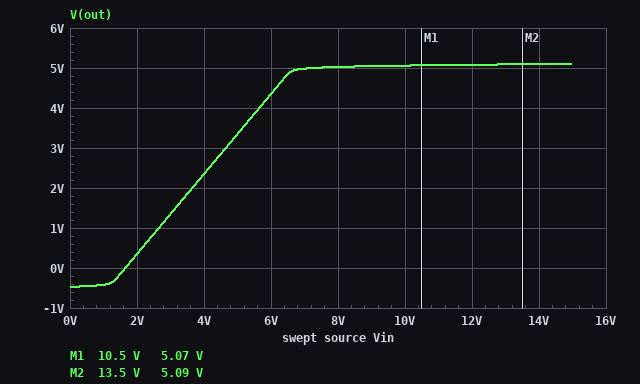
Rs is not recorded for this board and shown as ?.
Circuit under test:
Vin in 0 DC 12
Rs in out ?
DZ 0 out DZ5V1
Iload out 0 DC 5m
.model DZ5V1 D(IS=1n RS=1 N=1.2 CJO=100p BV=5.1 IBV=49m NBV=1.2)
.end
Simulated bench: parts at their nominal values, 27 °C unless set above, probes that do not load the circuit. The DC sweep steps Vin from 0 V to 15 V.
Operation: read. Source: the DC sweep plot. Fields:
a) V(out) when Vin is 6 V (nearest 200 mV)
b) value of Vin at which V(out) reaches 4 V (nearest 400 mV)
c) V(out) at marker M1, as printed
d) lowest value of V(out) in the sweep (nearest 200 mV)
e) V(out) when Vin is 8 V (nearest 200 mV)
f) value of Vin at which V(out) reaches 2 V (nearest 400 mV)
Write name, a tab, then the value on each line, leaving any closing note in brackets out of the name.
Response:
V(out) when Vin is 6 V	4.4 V
value of Vin at which V(out) reaches 4 V	5.6 V
V(out) at marker M1, as printed	5.07 V
lowest value of V(out) in the sweep	-400 mV
V(out) when Vin is 8 V	5.0 V
value of Vin at which V(out) reaches 2 V	3.6 V
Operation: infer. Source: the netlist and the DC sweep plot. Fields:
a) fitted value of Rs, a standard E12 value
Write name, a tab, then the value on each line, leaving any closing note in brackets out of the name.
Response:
fitted value of Rs, a standard E12 value	330 Ω
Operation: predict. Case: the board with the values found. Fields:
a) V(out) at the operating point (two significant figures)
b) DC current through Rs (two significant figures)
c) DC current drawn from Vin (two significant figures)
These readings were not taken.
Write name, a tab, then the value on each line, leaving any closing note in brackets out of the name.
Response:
V(out) at the operating point	5.1 V
DC current through Rs	21 mA
DC current drawn from Vin	21 mA
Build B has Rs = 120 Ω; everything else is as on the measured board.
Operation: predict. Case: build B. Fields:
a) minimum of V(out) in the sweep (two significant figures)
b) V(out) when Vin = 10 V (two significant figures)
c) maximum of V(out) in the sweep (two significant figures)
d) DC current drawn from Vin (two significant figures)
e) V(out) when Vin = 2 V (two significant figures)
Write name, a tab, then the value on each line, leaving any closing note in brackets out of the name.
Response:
minimum of V(out) in the sweep	-440 mV
V(out) when Vin = 10 V	5.1 V
maximum of V(out) in the sweep	5.2 V
DC current drawn from Vin	57 mA
V(out) when Vin = 2 V	1.4 V
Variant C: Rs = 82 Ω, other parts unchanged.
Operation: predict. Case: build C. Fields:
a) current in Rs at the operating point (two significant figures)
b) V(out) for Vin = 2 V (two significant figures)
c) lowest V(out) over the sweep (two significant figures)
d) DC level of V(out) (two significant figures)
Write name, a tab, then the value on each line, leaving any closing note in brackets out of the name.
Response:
current in Rs at the operating point	83 mA
V(out) for Vin = 2 V	1.6 V
lowest V(out) over the sweep	-390 mV
DC level of V(out)	5.2 V
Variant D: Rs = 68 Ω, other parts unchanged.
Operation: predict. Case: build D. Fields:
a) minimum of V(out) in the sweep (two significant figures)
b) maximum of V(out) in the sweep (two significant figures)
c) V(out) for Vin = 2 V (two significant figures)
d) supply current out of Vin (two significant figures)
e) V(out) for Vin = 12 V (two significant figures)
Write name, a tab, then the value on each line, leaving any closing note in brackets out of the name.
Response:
minimum of V(out) in the sweep	-340 mV
maximum of V(out) in the sweep	5.3 V
V(out) for Vin = 2 V	1.7 V
supply current out of Vin	100 mA
V(out) for Vin = 12 V	5.2 V
